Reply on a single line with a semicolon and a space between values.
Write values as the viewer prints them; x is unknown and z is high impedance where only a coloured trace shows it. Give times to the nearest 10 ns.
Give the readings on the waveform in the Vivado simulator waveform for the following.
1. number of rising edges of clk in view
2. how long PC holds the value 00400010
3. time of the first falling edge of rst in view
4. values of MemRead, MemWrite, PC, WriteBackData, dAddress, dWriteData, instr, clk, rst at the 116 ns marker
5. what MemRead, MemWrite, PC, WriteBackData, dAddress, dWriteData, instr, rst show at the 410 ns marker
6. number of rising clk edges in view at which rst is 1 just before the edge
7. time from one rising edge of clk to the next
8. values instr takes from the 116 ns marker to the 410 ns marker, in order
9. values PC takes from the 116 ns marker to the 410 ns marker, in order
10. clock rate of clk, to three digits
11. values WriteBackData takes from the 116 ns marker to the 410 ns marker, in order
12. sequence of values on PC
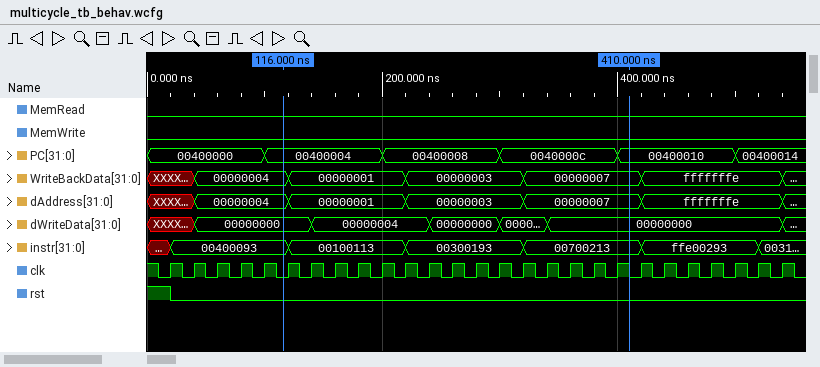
27; 100 ns; 20 ns; MemRead=0, MemWrite=0, PC=00400004, WriteBackData=00000004, dAddress=00000004, dWriteData=00000000, instr=00400093, clk=0, rst=0; MemRead=0, MemWrite=0, PC=00400010, WriteBackData=00000007, dAddress=00000007, dWriteData=00000000, instr=00700213, rst=0; 1; 20 ns; 00400093, 00100113, 00300193, 00700213; 00400004, 00400008, 0040000c, 00400010; 50.0 MHz; 00000004, 00000001, 00000003, 00000007; 00400000, 00400004, 00400008, 0040000c, 00400010, 00400014
